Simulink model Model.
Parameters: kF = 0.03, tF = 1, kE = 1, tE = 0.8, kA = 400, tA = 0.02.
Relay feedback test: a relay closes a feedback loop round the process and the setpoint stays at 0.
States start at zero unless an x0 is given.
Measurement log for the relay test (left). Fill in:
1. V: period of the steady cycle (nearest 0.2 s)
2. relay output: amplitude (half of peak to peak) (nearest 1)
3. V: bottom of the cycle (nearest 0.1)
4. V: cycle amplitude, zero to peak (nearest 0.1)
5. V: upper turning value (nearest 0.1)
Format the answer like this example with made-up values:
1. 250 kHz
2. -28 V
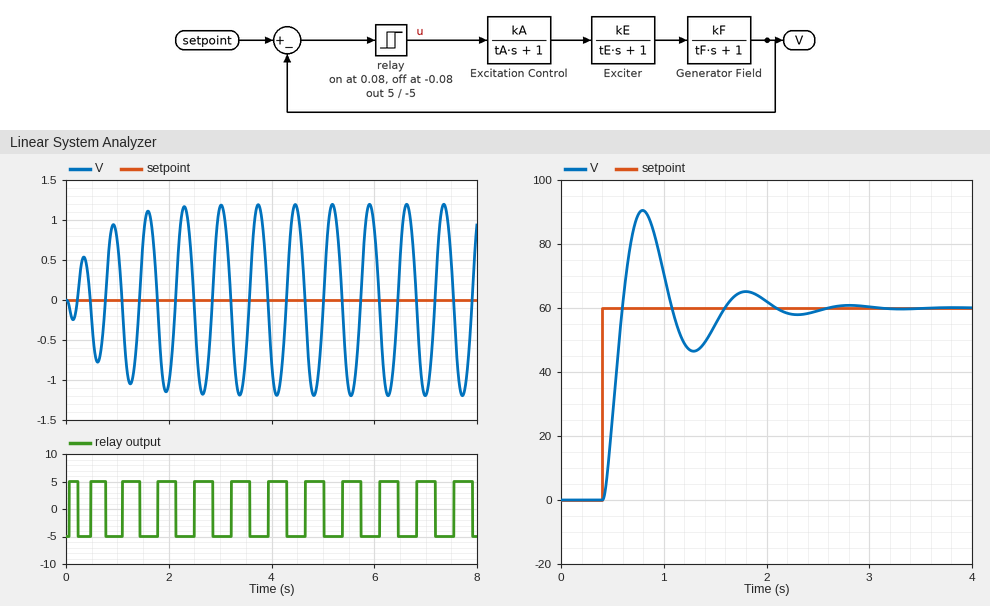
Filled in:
1. 0.8 s
2. 5
3. -1.2
4. 1.2
5. 1.2
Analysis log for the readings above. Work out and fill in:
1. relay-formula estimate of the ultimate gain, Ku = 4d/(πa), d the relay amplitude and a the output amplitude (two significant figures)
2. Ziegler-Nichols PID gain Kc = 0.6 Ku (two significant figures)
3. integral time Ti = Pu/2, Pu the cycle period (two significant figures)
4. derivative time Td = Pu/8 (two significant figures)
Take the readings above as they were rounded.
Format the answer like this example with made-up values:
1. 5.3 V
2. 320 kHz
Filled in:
1. 5.3
2. 3.2
3. 0.40 s
4. 0.10 s
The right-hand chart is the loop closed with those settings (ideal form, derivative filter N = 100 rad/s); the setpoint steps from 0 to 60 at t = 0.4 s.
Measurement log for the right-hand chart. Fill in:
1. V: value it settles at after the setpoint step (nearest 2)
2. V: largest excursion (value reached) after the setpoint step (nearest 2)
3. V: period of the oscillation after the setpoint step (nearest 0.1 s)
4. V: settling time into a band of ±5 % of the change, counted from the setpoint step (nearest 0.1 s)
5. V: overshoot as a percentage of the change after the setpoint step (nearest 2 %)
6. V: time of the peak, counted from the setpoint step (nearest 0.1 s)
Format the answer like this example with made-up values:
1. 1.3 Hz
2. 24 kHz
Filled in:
1. 60
2. 90
3. 1.0 s
4. 1.6 s
5. 50 %
6. 0.4 s
